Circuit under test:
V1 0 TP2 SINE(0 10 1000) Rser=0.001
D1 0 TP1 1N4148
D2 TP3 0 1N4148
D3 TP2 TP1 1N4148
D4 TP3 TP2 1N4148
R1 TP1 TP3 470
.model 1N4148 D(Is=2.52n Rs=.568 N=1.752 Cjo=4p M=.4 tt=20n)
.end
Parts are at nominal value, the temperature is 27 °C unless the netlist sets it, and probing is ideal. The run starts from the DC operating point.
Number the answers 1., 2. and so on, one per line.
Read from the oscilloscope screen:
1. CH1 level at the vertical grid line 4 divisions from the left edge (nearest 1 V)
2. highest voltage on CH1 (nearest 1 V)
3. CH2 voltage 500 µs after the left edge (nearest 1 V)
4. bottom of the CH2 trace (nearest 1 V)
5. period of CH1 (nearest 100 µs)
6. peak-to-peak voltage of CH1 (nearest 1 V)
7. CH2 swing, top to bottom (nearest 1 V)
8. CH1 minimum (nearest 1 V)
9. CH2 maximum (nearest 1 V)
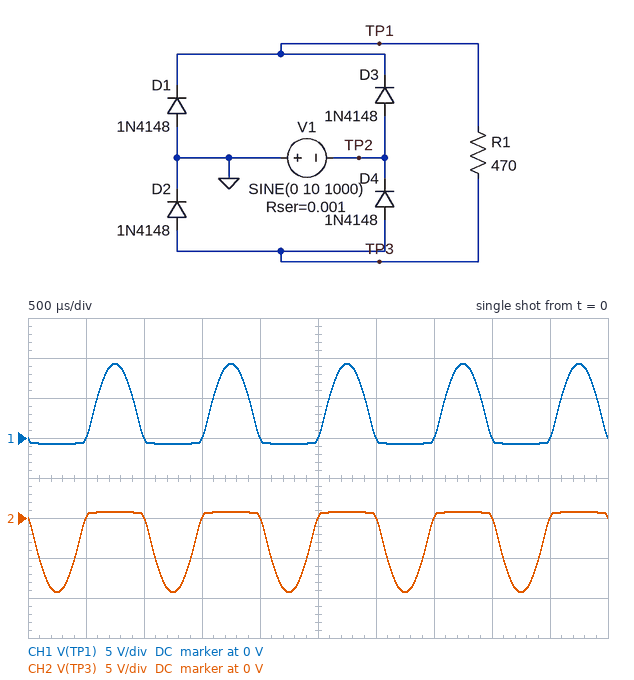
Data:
1. 0 V
2. 9 V
3. 0 V
4. -9 V
5. 1.0 ms
6. 10 V
7. 10 V
8. -1 V
9. 1 V
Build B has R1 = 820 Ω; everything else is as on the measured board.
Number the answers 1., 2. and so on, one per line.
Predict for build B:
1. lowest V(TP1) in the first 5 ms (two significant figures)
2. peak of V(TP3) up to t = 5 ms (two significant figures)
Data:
1. -700 mV
2. 700 mV
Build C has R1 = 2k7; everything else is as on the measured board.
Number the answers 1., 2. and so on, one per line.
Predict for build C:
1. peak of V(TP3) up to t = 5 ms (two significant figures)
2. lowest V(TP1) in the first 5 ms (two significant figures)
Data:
1. 640 mV
2. -640 mV
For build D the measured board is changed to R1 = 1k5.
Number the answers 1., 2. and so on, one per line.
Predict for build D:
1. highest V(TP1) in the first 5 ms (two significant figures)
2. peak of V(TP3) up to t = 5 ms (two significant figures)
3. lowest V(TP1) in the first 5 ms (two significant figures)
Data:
1. 9.3 V
2. 670 mV
3. -670 mV
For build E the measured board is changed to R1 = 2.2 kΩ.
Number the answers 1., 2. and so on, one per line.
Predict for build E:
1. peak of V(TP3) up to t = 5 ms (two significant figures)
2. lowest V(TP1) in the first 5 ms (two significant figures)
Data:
1. 650 mV
2. -650 mV
